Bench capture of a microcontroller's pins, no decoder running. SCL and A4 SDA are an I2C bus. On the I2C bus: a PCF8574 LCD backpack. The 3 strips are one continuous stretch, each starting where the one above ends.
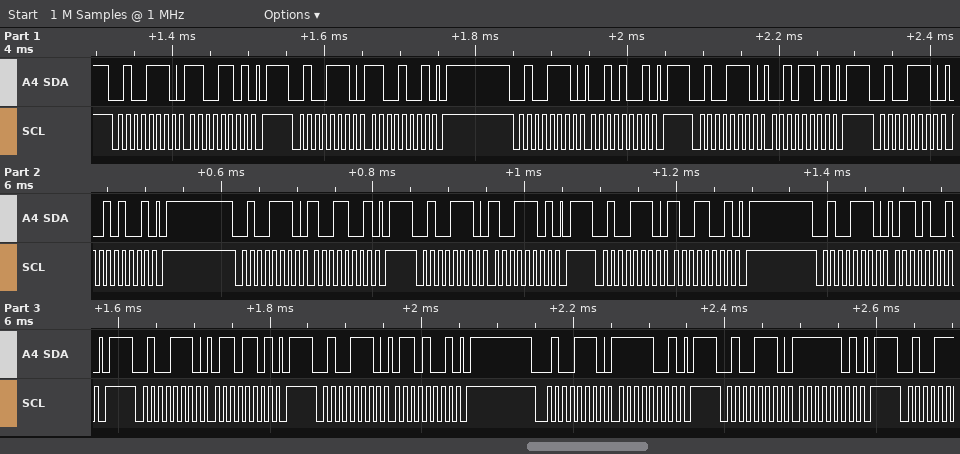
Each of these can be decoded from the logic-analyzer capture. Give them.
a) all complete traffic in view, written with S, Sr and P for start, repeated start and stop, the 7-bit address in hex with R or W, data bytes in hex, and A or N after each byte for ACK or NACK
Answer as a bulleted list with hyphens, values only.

- S 27W A CD A P S 27W A C9 A P S 27W A 29 A P S 27W A 2D A P S 27W A 29 A P S 27W A 99 A P S 27W A 9D A P S 27W A 99 A P S 27W A 69 A P S 27W A 6D A P S 27W A 69 A P S 27W A F9 A P S 27W A FD A P
